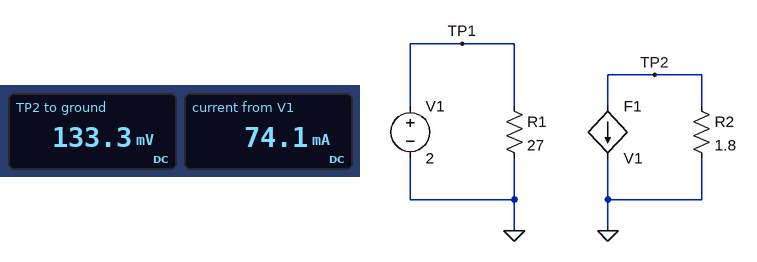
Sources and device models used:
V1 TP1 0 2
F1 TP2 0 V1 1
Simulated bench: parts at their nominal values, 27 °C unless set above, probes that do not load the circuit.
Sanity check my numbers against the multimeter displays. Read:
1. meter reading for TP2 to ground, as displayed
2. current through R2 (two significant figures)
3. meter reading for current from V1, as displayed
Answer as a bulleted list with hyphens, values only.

- 133.3 mV
- 74 mA
- 74.1 mA
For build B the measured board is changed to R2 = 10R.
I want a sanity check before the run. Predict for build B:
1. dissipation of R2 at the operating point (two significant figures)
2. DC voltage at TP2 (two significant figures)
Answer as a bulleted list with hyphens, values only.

- 55 mW
- 740 mV
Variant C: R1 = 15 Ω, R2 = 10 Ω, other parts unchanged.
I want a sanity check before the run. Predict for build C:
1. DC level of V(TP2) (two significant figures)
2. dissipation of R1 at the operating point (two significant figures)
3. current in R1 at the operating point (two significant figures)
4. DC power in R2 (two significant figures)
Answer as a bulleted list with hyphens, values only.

- 1.3 V
- 270 mW
- 130 mA
- 180 mW
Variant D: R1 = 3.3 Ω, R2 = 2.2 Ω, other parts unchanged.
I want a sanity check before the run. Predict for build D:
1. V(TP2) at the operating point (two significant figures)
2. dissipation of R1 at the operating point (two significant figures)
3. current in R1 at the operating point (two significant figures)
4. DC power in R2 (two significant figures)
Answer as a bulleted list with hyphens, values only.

- 1.3 V
- 1.2 W
- 610 mA
- 810 mW
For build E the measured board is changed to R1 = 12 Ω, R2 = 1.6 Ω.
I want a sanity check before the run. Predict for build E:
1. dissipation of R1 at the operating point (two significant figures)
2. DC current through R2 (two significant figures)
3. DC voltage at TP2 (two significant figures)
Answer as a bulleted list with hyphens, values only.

- 330 mW
- 170 mA
- 270 mV
